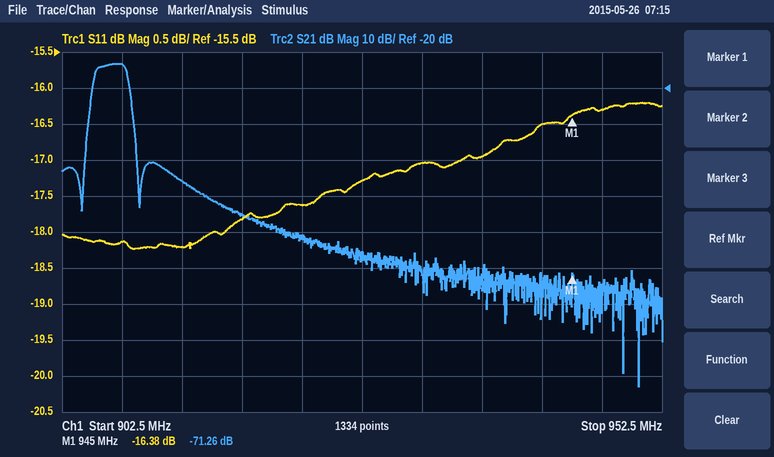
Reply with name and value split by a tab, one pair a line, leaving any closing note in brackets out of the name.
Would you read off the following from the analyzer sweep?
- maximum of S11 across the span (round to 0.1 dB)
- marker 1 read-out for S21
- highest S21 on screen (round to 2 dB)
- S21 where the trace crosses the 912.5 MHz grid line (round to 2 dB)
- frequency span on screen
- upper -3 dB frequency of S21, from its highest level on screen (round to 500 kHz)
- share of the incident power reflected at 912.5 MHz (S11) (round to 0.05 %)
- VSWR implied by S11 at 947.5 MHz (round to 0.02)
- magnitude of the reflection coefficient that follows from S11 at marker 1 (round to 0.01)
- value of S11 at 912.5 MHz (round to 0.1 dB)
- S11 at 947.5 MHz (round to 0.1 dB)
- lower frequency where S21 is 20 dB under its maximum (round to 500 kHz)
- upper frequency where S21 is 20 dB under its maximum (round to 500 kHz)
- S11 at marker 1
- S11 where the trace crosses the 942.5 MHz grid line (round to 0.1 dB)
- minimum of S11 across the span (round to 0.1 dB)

maximum of S11 across the span	-16.2 dB
marker 1 read-out for S21	-71.26 dB
highest S21 on screen	-14 dB
S21 where the trace crosses the 912.5 MHz grid line	-46 dB
frequency span on screen	50 MHz
upper -3 dB frequency of S21, from its highest level on screen	908.0 MHz
share of the incident power reflected at 912.5 MHz (S11)	1.50 %
VSWR implied by S11 at 947.5 MHz	1.36
magnitude of the reflection coefficient that follows from S11 at marker 1	0.15
value of S11 at 912.5 MHz	-18.2 dB
S11 at 947.5 MHz	-16.3 dB
lower frequency where S21 is 20 dB under its maximum	904.5 MHz
upper frequency where S21 is 20 dB under its maximum	908.5 MHz
S11 at marker 1	-16.38 dB
S11 where the trace crosses the 942.5 MHz grid line	-16.5 dB
minimum of S11 across the span	-18.2 dB
